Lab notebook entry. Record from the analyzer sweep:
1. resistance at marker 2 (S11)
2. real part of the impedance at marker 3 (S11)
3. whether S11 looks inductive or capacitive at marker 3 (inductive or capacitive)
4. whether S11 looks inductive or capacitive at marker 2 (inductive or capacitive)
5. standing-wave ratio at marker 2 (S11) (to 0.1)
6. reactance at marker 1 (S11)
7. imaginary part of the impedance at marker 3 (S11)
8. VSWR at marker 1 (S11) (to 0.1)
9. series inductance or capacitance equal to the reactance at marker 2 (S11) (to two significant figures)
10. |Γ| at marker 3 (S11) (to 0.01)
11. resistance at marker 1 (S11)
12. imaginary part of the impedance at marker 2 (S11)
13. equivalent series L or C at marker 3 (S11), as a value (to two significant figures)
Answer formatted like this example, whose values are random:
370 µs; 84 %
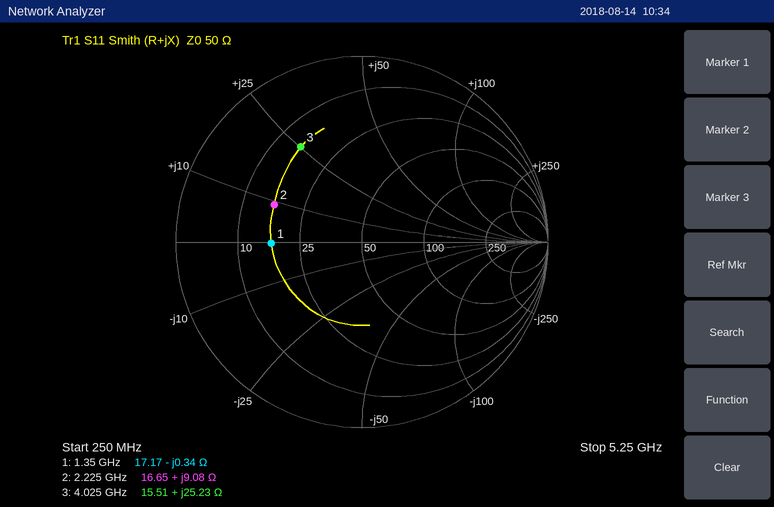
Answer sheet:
16.65 Ω; 15.51 Ω; inductive; inductive; 3.1; -0.34 Ω; +25.23 Ω; 2.9; 650 pH; 0.61; 17.17 Ω; +9.08 Ω; 1.00 nH
